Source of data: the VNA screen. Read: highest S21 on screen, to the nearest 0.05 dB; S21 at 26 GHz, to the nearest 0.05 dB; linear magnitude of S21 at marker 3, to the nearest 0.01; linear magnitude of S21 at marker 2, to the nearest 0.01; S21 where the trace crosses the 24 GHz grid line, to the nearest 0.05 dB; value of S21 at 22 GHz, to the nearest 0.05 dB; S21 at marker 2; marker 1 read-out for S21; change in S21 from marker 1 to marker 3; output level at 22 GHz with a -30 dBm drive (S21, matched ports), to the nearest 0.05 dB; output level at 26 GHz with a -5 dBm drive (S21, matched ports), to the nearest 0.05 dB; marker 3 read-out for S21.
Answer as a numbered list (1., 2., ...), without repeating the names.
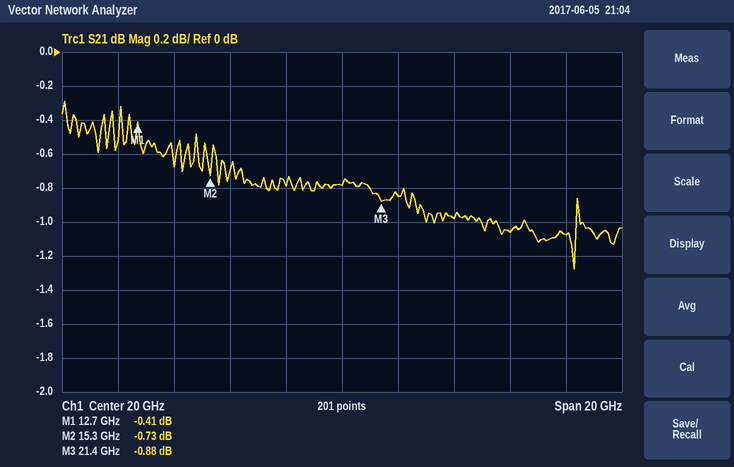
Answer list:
1. -0.30 dB
2. -1.05 dB
3. 0.90
4. 0.92
5. -1.00 dB
6. -0.85 dB
7. -0.73 dB
8. -0.41 dB
9. -0.47 dB
10. -30.85 dBm
11. -6.05 dBm
12. -0.88 dB
